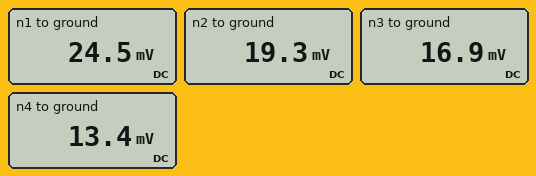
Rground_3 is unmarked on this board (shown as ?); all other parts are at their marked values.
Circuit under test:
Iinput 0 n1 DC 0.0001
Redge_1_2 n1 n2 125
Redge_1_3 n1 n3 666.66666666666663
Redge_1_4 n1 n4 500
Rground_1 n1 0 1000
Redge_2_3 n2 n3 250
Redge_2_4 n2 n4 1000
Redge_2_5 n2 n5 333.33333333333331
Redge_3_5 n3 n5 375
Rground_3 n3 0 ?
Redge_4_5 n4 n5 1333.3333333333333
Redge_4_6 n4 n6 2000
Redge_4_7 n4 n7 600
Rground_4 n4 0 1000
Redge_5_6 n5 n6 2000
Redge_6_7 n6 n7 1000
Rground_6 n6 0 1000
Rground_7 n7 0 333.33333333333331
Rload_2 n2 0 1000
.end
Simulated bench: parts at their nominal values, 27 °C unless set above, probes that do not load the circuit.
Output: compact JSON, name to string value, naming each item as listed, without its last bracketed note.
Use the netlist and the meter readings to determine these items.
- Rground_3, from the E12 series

{"Rground_3, from the E12 series": "820 Ω"}
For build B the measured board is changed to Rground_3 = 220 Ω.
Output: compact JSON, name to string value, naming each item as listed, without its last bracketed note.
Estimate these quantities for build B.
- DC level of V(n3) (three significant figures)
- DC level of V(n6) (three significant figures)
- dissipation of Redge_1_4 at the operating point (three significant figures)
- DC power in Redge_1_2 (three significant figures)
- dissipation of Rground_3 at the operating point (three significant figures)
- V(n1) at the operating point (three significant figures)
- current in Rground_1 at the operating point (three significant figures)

{"DC level of V(n3)": "8.91 mV", "DC level of V(n6)": "4.75 mV", "dissipation of Redge_1_4 at the operating point": "178 nW", "DC power in Redge_1_2": "262 nW", "dissipation of Rground_3 at the operating point": "361 nW", "V(n1) at the operating point": "19.5 mV", "current in Rground_1 at the operating point": "19.5 µA"}
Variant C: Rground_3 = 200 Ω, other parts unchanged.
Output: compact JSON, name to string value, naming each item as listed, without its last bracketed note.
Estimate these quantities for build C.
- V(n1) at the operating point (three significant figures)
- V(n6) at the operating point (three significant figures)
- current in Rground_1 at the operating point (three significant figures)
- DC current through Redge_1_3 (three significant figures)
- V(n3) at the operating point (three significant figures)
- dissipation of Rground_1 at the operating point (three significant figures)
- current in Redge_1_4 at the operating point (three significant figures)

{"V(n1) at the operating point": "19.2 mV", "V(n6) at the operating point": "4.62 mV", "current in Rground_1 at the operating point": "19.2 µA", "DC current through Redge_1_3": "16.2 µA", "V(n3) at the operating point": "8.37 mV", "dissipation of Rground_1 at the operating point": "367 nW", "current in Redge_1_4 at the operating point": "18.6 µA"}
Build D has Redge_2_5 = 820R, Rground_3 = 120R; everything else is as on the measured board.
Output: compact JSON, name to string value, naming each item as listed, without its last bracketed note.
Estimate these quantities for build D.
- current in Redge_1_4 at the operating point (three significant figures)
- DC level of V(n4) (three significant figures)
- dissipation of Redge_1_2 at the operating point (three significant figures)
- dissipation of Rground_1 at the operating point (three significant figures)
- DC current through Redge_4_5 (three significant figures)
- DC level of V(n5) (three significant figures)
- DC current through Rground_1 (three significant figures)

{"current in Redge_1_4 at the operating point": "18.1 µA", "DC level of V(n4)": "8.75 mV", "dissipation of Redge_1_2 at the operating point": "265 nW", "dissipation of Rground_1 at the operating point": "317 nW", "DC current through Redge_4_5": "948 nA", "DC level of V(n5)": "7.49 mV", "DC current through Rground_1": "17.8 µA"}
